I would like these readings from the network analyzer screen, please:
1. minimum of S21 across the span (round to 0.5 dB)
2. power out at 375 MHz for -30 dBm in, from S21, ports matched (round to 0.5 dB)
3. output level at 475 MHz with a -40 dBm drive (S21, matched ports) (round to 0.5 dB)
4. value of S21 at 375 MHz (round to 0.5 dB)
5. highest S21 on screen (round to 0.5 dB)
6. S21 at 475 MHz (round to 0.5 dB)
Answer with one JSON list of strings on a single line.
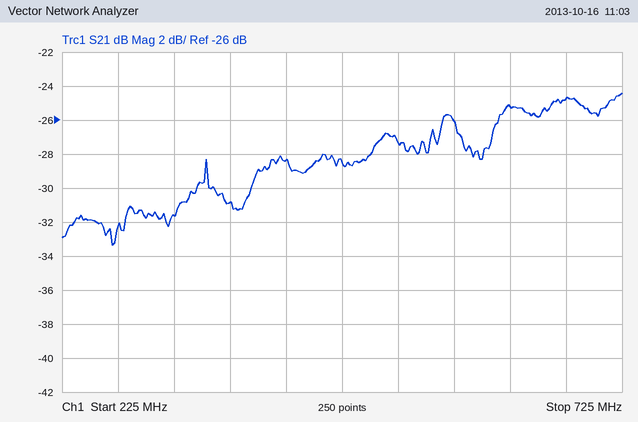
["-33.5 dB", "-61.0 dBm", "-68.5 dBm", "-31.0 dB", "-24.5 dB", "-28.5 dB"]
